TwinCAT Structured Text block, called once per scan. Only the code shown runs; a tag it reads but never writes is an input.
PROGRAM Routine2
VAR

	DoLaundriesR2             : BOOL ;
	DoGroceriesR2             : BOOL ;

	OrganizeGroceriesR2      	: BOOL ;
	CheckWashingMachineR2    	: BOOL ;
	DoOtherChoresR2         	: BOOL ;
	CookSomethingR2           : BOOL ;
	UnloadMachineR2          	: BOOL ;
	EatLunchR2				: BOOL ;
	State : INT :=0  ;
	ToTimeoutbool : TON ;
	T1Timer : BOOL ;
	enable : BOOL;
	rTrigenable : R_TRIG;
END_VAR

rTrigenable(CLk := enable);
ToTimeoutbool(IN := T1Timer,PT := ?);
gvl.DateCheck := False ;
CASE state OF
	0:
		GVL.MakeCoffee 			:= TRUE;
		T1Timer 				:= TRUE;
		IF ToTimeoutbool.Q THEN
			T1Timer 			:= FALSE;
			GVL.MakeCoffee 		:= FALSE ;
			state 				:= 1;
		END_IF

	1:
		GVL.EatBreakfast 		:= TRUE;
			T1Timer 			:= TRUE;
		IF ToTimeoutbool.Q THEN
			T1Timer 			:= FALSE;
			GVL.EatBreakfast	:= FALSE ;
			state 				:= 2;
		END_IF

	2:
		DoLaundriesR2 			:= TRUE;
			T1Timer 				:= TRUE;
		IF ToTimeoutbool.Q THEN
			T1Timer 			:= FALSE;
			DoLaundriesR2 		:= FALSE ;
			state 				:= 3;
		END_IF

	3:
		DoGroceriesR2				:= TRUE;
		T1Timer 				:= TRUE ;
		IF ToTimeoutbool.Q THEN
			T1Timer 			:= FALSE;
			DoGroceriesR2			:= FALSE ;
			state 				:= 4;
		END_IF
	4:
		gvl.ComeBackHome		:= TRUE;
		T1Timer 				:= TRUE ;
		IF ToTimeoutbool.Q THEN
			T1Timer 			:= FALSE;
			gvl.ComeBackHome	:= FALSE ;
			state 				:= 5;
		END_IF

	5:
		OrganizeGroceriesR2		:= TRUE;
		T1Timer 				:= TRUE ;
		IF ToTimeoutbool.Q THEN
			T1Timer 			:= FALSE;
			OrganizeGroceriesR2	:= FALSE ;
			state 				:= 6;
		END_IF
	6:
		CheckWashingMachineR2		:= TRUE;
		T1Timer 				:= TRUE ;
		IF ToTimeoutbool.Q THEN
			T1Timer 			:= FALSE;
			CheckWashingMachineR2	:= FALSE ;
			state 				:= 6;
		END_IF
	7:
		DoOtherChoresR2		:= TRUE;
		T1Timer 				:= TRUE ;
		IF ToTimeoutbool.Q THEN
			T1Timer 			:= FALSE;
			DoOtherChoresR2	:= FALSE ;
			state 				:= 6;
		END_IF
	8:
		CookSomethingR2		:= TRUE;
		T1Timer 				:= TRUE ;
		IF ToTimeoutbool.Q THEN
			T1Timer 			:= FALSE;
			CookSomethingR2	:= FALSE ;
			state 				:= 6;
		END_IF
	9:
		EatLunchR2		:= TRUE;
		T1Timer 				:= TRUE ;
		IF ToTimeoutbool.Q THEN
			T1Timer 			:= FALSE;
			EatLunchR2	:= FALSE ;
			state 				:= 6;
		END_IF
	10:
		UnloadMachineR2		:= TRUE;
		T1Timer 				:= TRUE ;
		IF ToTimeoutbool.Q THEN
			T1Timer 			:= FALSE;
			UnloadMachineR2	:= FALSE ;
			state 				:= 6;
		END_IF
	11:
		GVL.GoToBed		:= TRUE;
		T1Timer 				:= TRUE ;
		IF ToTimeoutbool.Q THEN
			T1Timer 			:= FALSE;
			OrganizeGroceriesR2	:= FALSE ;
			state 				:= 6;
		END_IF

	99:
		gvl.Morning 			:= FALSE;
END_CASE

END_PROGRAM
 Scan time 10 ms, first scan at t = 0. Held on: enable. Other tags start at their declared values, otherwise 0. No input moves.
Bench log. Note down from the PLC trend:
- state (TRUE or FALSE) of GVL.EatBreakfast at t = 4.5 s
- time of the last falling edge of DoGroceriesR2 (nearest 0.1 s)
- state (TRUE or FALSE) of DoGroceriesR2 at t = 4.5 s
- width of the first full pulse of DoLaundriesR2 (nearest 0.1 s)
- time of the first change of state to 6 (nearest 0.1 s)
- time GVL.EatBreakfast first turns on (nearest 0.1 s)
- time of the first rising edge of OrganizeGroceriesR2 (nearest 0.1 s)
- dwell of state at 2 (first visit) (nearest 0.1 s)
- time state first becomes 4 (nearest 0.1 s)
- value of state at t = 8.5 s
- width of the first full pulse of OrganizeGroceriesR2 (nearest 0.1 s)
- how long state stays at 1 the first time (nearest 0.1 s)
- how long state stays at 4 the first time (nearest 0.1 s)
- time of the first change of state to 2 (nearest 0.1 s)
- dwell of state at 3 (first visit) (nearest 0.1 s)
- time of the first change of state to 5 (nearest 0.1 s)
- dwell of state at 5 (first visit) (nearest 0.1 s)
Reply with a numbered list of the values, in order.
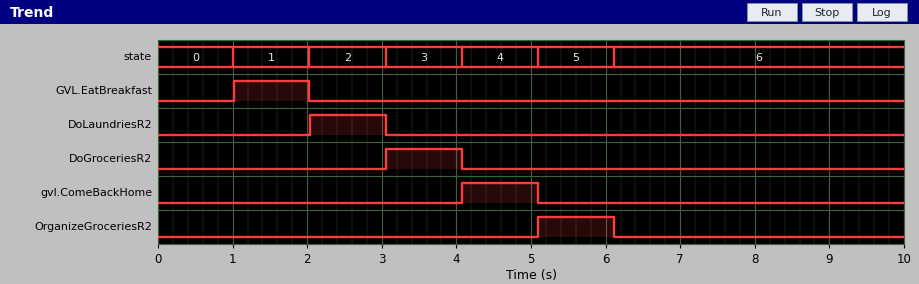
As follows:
1. FALSE
2. 4.1 s
3. FALSE
4. 1.0 s
5. 6.1 s
6. 1.0 s
7. 5.1 s
8. 1.0 s
9. 4.1 s
10. 6
11. 1.0 s
12. 1.0 s
13. 1.0 s
14. 2.0 s
15. 1.0 s
16. 5.1 s
17. 1.0 s
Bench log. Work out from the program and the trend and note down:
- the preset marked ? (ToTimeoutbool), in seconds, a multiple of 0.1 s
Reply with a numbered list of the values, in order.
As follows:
1. 1.0 s
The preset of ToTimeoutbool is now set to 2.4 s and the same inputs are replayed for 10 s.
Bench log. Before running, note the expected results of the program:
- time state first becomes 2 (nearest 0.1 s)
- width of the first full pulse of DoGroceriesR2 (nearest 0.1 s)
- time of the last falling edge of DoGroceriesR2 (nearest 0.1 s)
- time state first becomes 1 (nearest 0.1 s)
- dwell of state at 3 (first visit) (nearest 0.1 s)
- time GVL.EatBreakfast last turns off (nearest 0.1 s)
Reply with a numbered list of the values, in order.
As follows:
1. 4.8 s
2. 2.4 s
3. 9.7 s
4. 2.4 s
5. 2.4 s
6. 4.8 s
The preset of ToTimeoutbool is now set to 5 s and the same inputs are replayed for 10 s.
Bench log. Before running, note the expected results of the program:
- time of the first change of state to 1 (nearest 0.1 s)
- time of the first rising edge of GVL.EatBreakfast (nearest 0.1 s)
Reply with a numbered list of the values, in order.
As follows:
1. 5.0 s
2. 5.0 s
